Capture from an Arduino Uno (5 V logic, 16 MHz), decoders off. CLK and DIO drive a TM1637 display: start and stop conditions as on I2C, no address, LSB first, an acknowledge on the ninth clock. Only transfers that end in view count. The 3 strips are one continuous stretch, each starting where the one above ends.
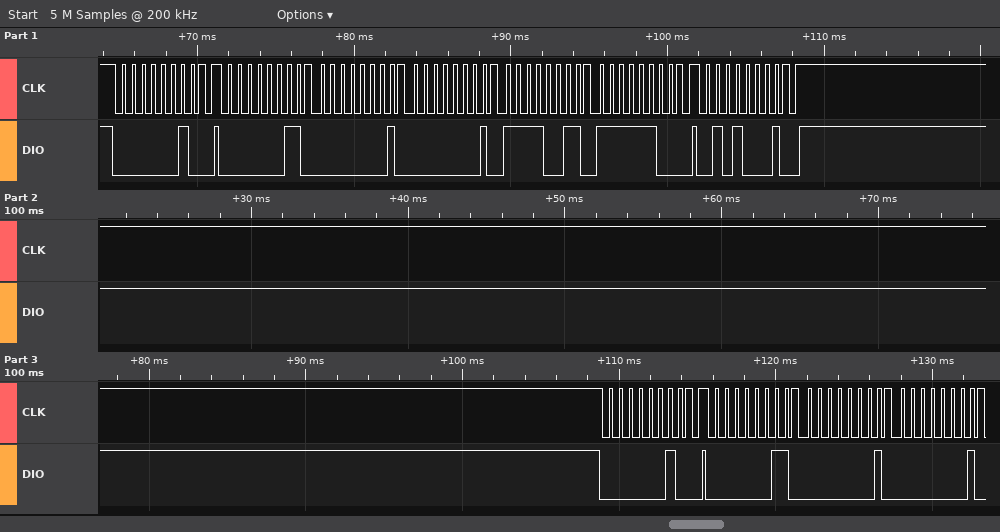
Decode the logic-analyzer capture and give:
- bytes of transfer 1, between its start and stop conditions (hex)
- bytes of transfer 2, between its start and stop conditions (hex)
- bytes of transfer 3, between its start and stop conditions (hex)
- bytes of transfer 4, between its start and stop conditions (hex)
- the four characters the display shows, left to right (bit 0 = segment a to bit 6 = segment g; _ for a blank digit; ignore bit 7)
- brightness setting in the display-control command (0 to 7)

40
C0 80 80 CF 3F
8A
40
__30
2
